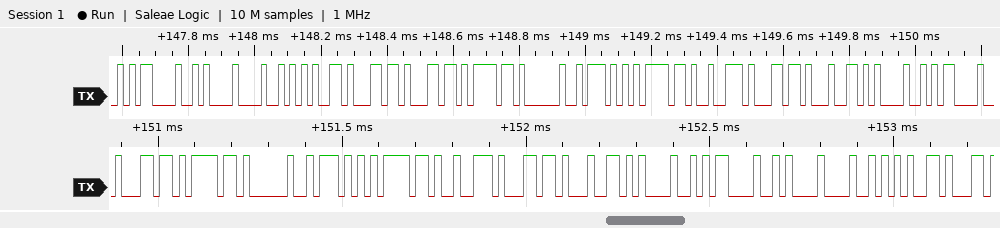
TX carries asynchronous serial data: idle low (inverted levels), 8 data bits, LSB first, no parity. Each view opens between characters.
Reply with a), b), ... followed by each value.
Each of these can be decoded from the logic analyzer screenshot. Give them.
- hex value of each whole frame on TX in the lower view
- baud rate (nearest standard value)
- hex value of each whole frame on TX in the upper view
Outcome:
a) 27, 21, BF, 51, 21, 1B, 27, 37, BD, E5, EB, 6F, 35
b) 57600 baud
c) E5, EB, 6F, 35, 27, 27, 21, BF, 51, 21, 1B, 27, 37, BD, E5
